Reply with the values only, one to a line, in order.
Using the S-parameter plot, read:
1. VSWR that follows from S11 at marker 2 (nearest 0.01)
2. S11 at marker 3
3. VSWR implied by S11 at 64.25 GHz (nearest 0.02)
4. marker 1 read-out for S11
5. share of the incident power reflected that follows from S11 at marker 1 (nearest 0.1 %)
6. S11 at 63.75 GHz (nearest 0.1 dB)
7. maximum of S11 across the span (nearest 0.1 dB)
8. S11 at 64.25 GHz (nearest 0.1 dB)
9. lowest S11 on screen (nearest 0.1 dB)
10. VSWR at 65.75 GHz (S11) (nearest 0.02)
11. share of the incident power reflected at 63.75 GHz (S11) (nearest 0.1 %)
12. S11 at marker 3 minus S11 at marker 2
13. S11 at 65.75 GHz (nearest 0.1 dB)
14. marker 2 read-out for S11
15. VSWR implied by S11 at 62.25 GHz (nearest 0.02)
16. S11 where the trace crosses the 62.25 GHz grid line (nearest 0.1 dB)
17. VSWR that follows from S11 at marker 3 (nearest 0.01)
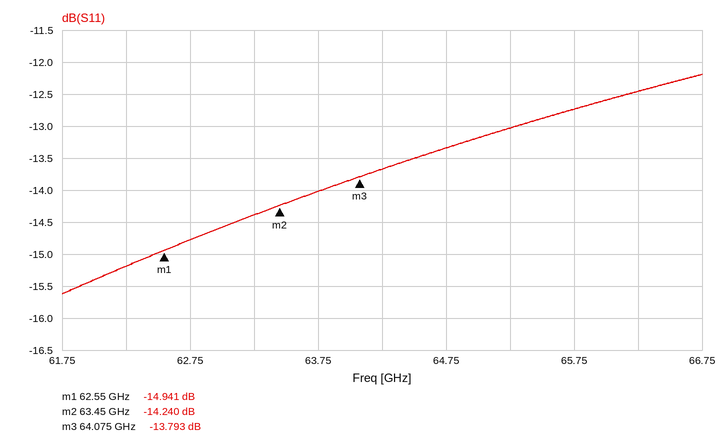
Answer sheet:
1.48
-13.793 dB
1.52
-14.941 dB
3.2 %
-14.0 dB
-12.2 dB
-13.7 dB
-15.6 dB
1.60
4.0 %
0.447 dB
-12.7 dB
-14.240 dB
1.42
-15.2 dB
1.51
